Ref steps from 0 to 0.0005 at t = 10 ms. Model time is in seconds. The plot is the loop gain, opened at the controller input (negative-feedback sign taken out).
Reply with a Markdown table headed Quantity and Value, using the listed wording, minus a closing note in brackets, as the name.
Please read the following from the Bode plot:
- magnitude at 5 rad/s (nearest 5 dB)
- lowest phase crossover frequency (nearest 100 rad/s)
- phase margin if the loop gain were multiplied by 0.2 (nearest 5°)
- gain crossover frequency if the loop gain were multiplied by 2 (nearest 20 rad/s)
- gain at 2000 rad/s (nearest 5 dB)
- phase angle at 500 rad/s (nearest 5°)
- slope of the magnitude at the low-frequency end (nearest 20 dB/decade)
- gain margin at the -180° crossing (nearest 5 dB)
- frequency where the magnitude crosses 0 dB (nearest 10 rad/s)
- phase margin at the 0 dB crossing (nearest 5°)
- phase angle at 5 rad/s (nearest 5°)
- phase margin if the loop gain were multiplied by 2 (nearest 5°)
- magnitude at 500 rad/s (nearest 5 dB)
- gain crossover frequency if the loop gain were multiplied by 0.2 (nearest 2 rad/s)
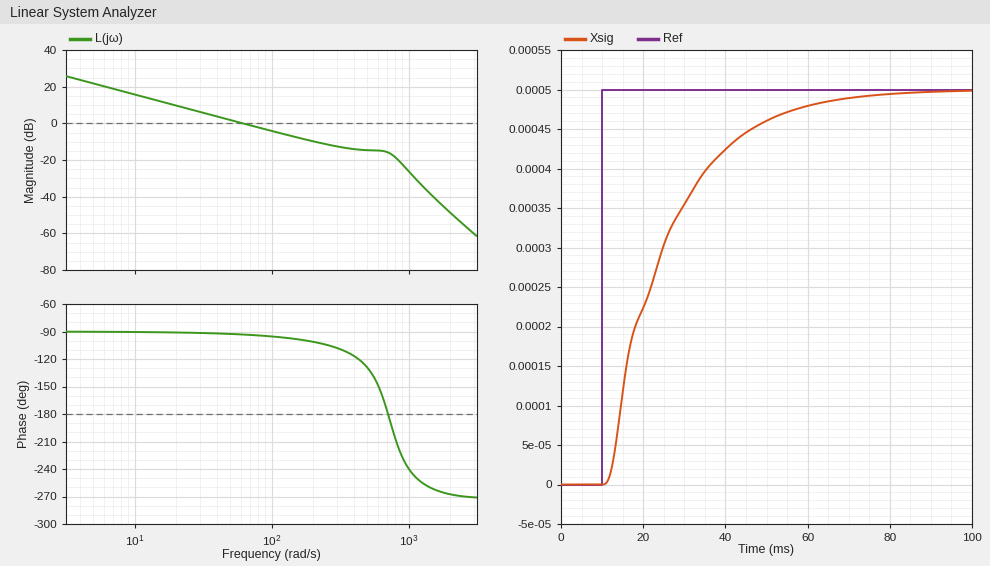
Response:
| Quantity | Value |
|---|---|
| magnitude at 5 rad/s | 20 dB |
| lowest phase crossover frequency | 700 rad/s |
| phase margin if the loop gain were multiplied by 0.2 | 90° |
| gain crossover frequency if the loop gain were multiplied by 2 | 120 rad/s |
| gain at 2000 rad/s | -50 dB |
| phase angle at 500 rad/s | -130° |
| slope of the magnitude at the low-frequency end | -20 dB/decade |
| gain margin at the -180° crossing | 15 dB |
| frequency where the magnitude crosses 0 dB | 60 rad/s |
| phase margin at the 0 dB crossing | 85° |
| phase angle at 5 rad/s | -90° |
| phase margin if the loop gain were multiplied by 2 | 85° |
| magnitude at 500 rad/s | -15 dB |
| gain crossover frequency if the loop gain were multiplied by 0.2 | 12 rad/s |
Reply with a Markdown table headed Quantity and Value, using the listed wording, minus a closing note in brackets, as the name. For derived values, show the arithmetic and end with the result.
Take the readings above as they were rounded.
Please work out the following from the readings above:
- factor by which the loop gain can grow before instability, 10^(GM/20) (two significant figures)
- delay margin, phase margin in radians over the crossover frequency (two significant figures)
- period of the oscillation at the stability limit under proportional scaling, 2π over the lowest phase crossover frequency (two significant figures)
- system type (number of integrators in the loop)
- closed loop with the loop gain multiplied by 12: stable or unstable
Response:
| Quantity | Value |
|---|---|
| factor by which the loop gain can grow before instability, 10^(GM/20) | 10^(15 / 20) = 5.6 |
| delay margin, phase margin in radians over the crossover frequency | 85 × π / 180 / 60 = 0.025 s |
| period of the oscillation at the stability limit under proportional scaling, 2π over the lowest phase crossover frequency | 2π / 700 = 0.0090 s |
| system type | 1 |
| closed loop with the loop gain multiplied by 12: stable or unstable | unstable |
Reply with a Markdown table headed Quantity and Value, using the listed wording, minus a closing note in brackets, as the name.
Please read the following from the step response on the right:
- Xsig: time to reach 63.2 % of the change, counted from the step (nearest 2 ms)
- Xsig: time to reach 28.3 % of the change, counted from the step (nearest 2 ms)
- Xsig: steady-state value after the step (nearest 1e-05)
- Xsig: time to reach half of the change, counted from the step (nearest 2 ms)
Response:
| Quantity | Value |
|---|---|
| Xsig: time to reach 63.2 % of the change, counted from the step | 16 ms |
| Xsig: time to reach 28.3 % of the change, counted from the step | 6 ms |
| Xsig: steady-state value after the step | 0.00050 |
| Xsig: time to reach half of the change, counted from the step | 12 ms |
